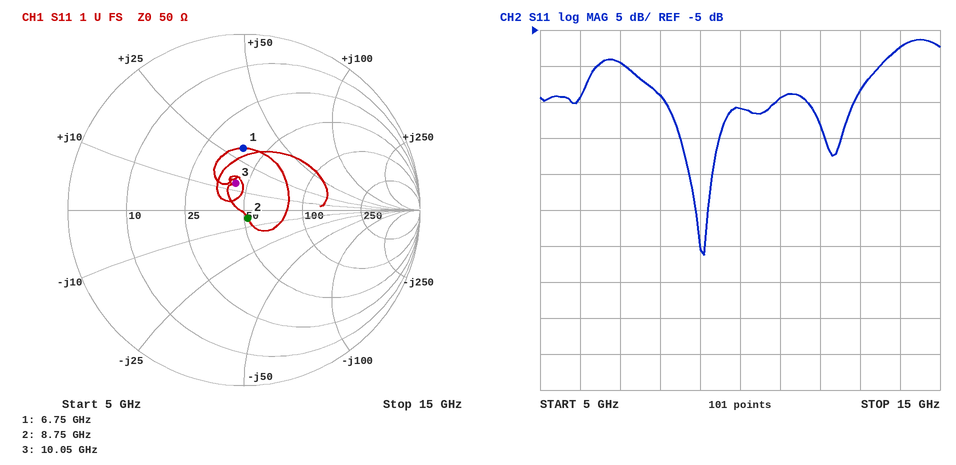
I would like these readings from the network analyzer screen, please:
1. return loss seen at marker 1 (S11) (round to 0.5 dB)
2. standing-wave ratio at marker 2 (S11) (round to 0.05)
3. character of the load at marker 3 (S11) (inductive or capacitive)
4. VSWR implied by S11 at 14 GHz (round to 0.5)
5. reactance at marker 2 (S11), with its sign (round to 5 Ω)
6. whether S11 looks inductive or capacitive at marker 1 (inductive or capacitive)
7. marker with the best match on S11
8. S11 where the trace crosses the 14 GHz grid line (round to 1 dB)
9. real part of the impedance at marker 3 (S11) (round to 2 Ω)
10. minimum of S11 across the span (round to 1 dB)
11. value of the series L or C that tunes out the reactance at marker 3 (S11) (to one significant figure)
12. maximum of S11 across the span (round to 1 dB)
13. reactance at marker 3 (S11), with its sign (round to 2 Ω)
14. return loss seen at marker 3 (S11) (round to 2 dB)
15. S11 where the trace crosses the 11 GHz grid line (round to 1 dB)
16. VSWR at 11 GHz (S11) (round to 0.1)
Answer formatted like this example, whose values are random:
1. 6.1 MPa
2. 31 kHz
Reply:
1. 9.0 dB
2. 1.10
3. inductive
4. 2.5
5. -5 Ω
6. inductive
7. marker 2
8. -7 dB
9. 44 Ω
10. -36 dB
11. 1 pF
12. -6 dB
13. +14 Ω
14. 16 dB
15. -14 dB
16. 1.5
